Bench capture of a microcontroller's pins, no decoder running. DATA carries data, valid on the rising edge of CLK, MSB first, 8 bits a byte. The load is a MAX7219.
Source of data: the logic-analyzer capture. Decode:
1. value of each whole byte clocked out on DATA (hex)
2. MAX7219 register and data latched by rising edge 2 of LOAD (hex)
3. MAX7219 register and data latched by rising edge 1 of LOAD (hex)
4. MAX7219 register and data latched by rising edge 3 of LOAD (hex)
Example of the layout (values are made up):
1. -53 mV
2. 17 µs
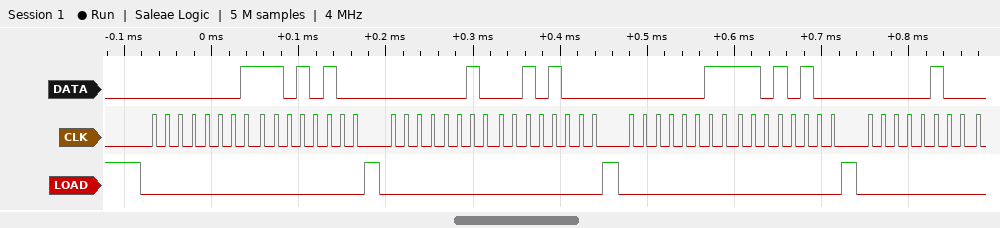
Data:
1. 01 D4 02 28 03 D4 04
2. register 0x2, data 0x28
3. register 0x1, data 0xD4
4. register 0x3, data 0xD4
